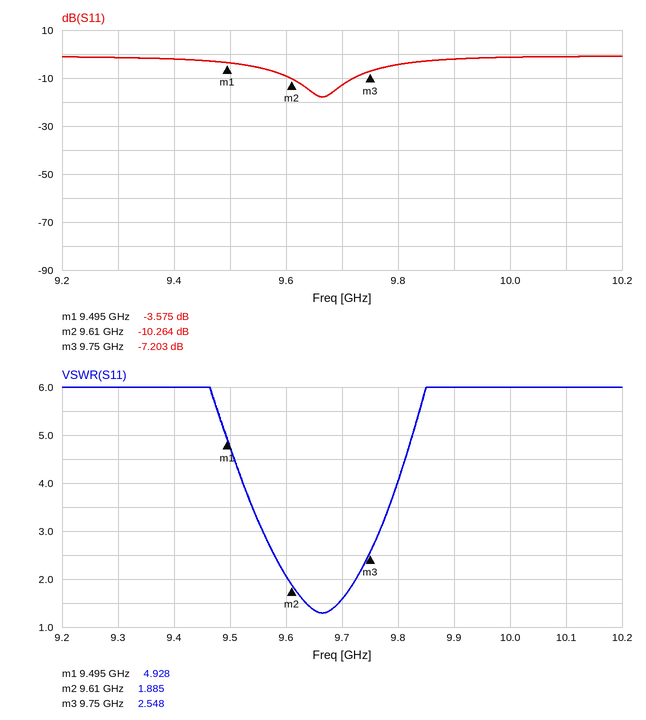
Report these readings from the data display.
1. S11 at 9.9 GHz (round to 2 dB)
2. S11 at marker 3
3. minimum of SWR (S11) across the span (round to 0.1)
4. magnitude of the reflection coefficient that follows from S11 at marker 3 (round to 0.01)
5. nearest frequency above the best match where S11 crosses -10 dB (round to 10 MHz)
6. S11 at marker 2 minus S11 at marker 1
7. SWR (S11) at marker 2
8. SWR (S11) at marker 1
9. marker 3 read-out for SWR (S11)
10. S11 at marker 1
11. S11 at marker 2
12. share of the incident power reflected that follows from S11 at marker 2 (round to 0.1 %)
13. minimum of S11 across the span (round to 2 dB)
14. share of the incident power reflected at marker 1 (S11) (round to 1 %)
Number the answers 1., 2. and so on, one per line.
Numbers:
1. -2 dB
2. -7.203 dB
3. 1.3
4. 0.44
5. 9.72 GHz
6. -6.689 dB
7. 1.885
8. 4.928
9. 2.548
10. -3.575 dB
11. -10.264 dB
12. 9.4 %
13. -18 dB
14. 44 %
